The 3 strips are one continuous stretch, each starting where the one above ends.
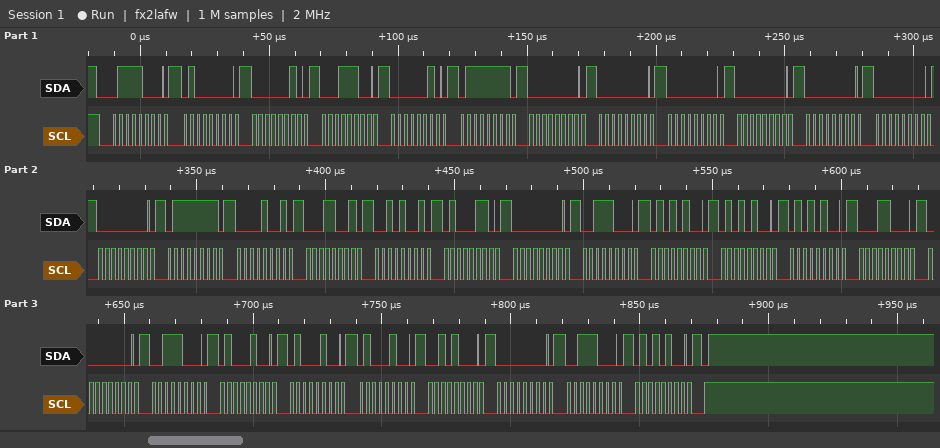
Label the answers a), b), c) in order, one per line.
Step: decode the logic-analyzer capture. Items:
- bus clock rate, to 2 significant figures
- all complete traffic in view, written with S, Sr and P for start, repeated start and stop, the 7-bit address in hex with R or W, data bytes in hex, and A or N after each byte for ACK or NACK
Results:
a) 400 kHz
b) S 3CW A 40 A 02 A 1C A 02 A 7F A 00 A 00 A 00 A 00 A 00 A 00 A 00 A 7F A 09 A 19 A 29 A 46 A 00 A 38 A 54 A 54 A 54 A 18 A 00 A 38 A 44 A 44 A 44 A 28 A 00 A 38 A 54 A P
